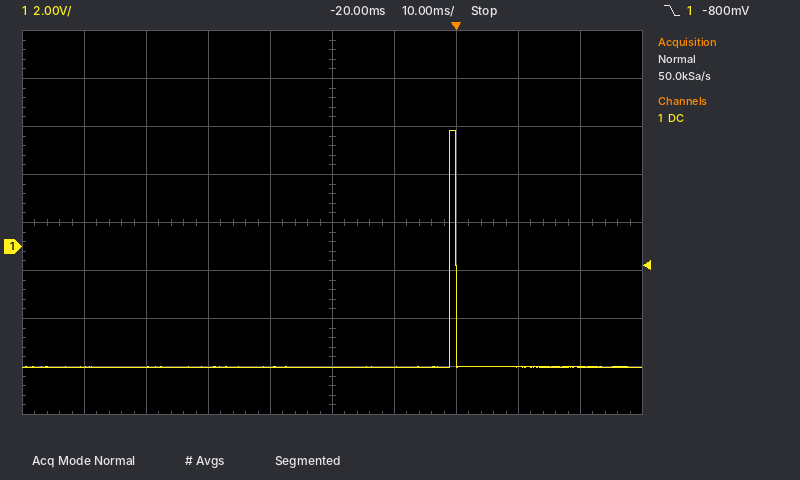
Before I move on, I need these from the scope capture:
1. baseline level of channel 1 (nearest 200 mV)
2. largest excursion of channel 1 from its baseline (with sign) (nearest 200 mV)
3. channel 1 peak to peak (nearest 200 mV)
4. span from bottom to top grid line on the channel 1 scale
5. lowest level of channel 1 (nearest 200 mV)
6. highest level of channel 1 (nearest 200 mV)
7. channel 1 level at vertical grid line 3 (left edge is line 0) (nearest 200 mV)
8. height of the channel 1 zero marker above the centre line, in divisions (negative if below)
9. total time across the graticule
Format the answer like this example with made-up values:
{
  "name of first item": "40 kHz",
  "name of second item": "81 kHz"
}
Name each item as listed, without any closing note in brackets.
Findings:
{
  "baseline level of channel 1": "-5.0 V",
  "largest excursion of channel 1 from its baseline (with sign)": "+9.8 V",
  "channel 1 peak to peak": "9.8 V",
  "span from bottom to top grid line on the channel 1 scale": "16 V",
  "lowest level of channel 1": "-5.0 V",
  "highest level of channel 1": "4.8 V",
  "channel 1 level at vertical grid line 3 (left edge is line 0)": "-5.0 V",
  "height of the channel 1 zero marker above the centre line, in divisions": "-0.5 div",
  "total time across the graticule": "100 ms"
}
